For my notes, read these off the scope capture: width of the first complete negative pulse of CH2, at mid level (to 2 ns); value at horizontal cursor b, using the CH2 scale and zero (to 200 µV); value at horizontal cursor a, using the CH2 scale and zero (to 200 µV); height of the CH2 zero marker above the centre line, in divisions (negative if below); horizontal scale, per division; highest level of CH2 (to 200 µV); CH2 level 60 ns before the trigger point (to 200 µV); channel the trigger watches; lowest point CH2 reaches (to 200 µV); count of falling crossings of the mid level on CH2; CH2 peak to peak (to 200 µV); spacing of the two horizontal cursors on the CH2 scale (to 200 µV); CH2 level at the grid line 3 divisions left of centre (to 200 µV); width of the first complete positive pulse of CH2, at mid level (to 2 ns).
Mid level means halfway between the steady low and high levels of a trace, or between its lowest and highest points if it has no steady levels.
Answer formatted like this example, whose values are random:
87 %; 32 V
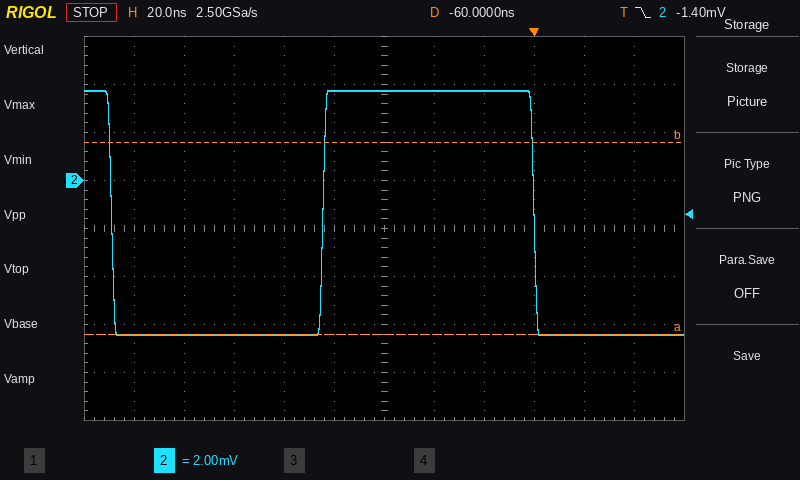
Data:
84 ns; 1.6 mV; -6.4 mV; +1.0 div; 20 ns; 3.8 mV; 3.8 mV; CH2; -6.4 mV; 2; 10.2 mV; 8.0 mV; -6.4 mV; 84 ns
